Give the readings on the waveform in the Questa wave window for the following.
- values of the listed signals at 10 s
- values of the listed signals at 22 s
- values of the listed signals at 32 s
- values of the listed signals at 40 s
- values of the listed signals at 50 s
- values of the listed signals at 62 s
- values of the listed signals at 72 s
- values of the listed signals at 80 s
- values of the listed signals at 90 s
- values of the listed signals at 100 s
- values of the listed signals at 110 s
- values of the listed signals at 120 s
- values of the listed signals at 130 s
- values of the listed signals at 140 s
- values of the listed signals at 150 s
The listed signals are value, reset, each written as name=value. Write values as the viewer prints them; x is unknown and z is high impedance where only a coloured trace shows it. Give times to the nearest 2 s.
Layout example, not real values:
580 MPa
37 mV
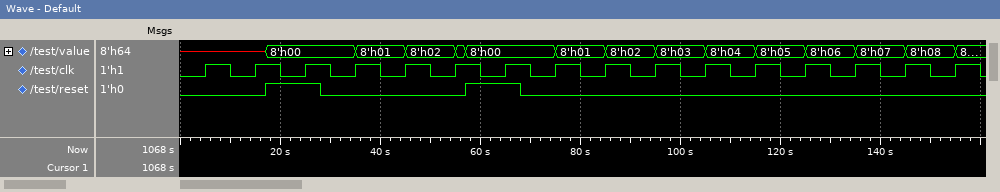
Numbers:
value=x, reset=0
value=8'h00, reset=1
value=8'h00, reset=0
value=8'h01, reset=0
value=8'h02, reset=0
value=8'h00, reset=1
value=8'h00, reset=0
value=8'h01, reset=0
value=8'h02, reset=0
value=8'h03, reset=0
value=8'h04, reset=0
value=8'h05, reset=0
value=8'h06, reset=0
value=8'h07, reset=0
value=8'h08, reset=0
